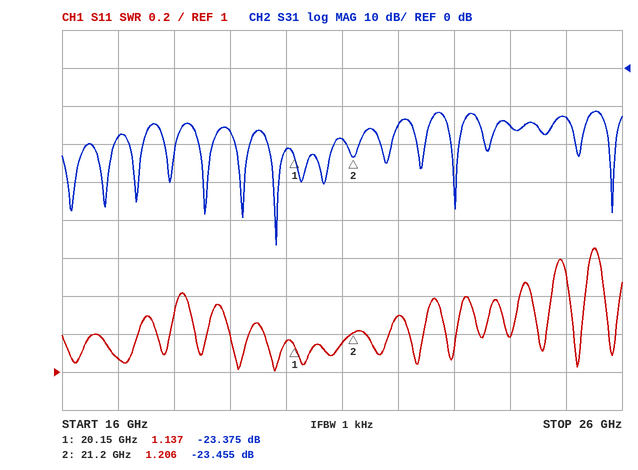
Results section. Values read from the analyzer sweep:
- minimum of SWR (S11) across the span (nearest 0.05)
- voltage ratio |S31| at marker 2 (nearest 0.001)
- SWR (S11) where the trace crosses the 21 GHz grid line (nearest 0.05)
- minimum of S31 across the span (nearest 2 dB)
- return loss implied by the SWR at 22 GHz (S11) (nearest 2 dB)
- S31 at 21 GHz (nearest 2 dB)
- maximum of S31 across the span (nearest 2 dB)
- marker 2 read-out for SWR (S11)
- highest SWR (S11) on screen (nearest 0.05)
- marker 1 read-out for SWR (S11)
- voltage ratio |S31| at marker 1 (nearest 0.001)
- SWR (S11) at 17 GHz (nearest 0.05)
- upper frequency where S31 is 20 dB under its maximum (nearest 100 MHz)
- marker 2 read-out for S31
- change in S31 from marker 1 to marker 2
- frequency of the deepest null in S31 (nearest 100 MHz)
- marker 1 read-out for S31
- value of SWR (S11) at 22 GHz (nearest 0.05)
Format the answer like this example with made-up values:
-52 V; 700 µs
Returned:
1.00; 0.067; 1.15; -46 dB; 18 dB; -18 dB; -12 dB; 1.206; 1.65; 1.137; 0.068; 1.05; 25.8 GHz; -23.455 dB; -0.080 dB; 19.8 GHz; -23.375 dB; 1.30
